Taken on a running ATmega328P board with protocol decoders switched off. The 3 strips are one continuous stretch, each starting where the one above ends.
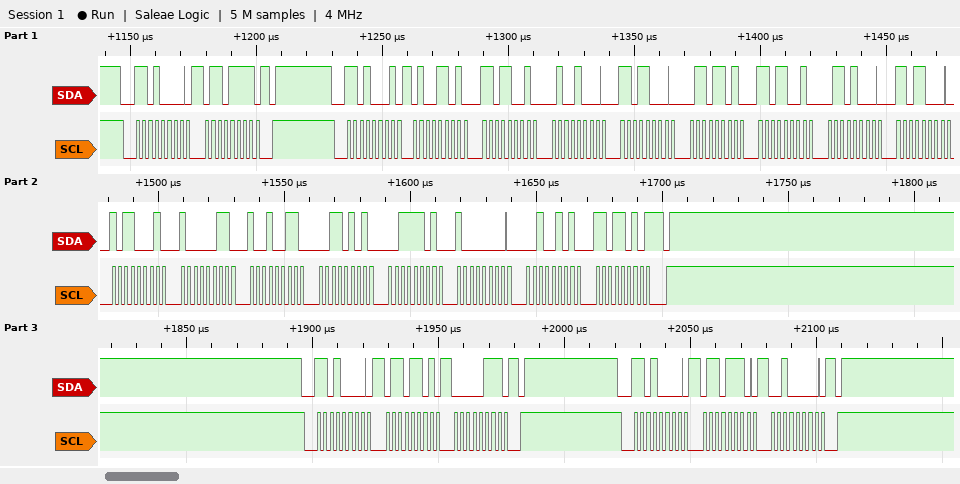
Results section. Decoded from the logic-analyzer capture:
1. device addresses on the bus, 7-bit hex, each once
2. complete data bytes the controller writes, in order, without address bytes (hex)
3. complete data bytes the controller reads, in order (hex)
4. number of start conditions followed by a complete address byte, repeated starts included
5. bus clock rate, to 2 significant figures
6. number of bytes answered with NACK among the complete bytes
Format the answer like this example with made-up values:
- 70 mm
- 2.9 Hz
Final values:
- 0x68
- 6F 6D 07 6E 20
- 4D D9 48 D8 6D D9 68 D8 B1 83 93 35 3D 80 25 DA
- 4
- 400 kHz
- 1
